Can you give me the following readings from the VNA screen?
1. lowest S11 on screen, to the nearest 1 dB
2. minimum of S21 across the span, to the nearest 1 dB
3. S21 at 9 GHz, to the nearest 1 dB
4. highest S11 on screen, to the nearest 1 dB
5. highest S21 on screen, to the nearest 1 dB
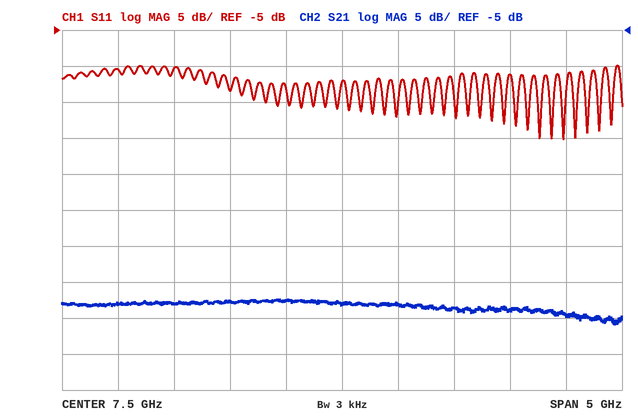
-20 dB
-46 dB
-44 dB
-10 dB
-42 dB
